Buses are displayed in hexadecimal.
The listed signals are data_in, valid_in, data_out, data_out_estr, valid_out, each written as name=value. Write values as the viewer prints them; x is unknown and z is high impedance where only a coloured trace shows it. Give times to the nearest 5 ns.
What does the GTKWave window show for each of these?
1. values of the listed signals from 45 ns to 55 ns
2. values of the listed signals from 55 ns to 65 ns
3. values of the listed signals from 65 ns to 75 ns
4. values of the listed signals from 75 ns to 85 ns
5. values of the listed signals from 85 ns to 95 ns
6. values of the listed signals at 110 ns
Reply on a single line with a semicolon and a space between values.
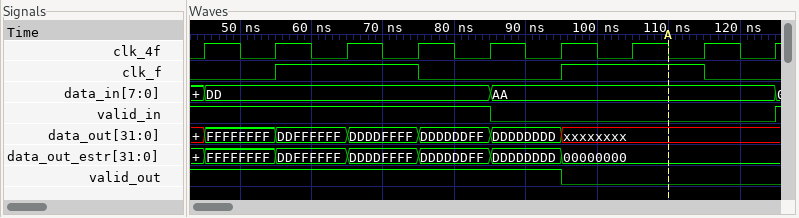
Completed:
data_in=DD, valid_in=1, data_out=FFFFFFFF, data_out_estr=FFFFFFFF, valid_out=1; data_in=DD, valid_in=1, data_out=DDFFFFFF, data_out_estr=DDFFFFFF, valid_out=1; data_in=DD, valid_in=1, data_out=DDDDFFFF, data_out_estr=DDDDFFFF, valid_out=1; data_in=DD, valid_in=1, data_out=DDDDDDFF, data_out_estr=DDDDDDFF, valid_out=1; data_in=AA, valid_in=0, data_out=DDDDDDDD, data_out_estr=DDDDDDDD, valid_out=1; data_in=AA, valid_in=0, data_out=xxxxxxxx, data_out_estr=00000000, valid_out=0
